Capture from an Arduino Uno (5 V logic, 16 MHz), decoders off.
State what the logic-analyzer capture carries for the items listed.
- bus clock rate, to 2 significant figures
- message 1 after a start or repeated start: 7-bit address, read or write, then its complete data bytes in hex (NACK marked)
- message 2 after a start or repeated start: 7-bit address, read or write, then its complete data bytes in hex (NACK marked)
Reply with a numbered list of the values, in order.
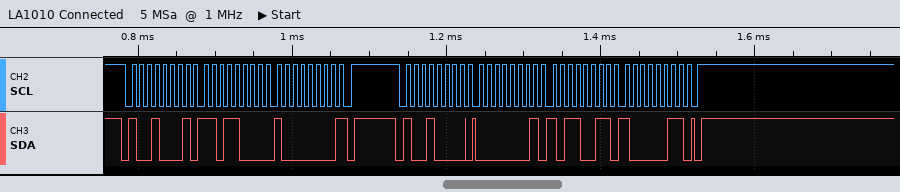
1. 100 kHz
2. 0x48 read: D8 80 NACK
3. 0x48 write: 01 B3 83
